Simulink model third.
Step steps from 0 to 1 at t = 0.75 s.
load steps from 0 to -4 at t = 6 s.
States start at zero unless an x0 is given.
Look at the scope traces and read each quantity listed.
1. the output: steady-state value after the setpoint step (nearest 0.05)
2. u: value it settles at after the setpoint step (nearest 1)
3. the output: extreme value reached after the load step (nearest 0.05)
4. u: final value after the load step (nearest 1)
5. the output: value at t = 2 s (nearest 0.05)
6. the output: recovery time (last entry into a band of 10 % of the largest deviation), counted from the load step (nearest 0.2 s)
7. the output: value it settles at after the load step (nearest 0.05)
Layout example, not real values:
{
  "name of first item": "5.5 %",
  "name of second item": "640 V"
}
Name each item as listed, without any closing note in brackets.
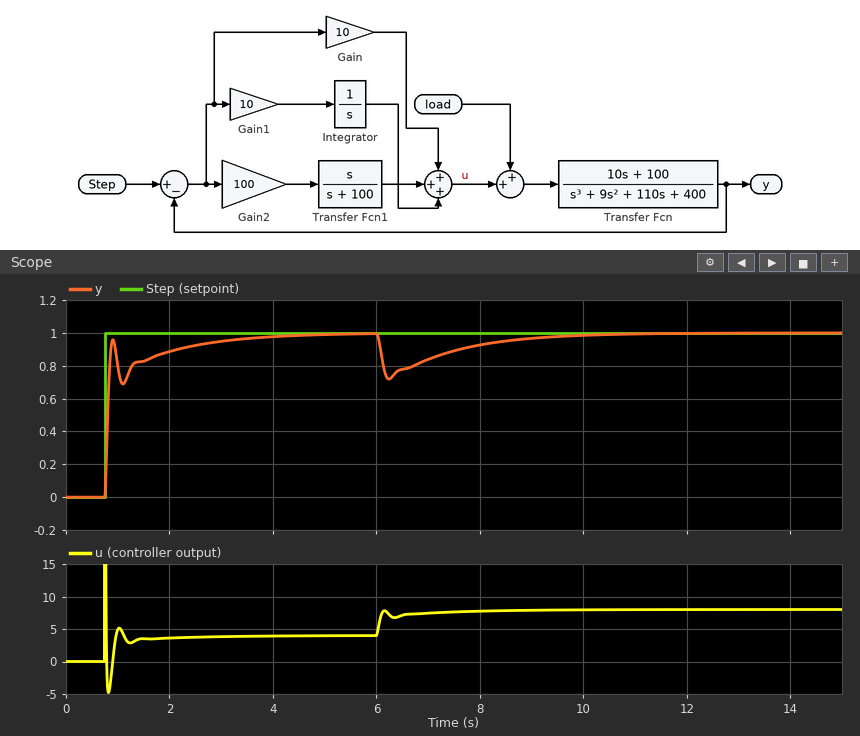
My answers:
{
  "the output: steady-state value after the setpoint step": "1.00",
  "u: value it settles at after the setpoint step": "4",
  "the output: extreme value reached after the load step": "0.70",
  "u: final value after the load step": "8",
  "the output: value at t = 2 s": "0.90",
  "the output: recovery time (last entry into a band of 10 % of the largest deviation), counted from the load step": "3.2 s",
  "the output: value it settles at after the load step": "1.00"
}
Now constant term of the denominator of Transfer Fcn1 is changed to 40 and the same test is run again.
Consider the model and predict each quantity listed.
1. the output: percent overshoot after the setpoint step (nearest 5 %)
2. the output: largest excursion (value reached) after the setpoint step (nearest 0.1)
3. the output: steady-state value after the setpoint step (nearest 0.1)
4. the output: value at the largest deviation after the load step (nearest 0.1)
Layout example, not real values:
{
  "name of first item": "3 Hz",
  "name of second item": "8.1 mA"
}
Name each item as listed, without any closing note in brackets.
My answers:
{
  "the output: percent overshoot after the setpoint step": "10 %",
  "the output: largest excursion (value reached) after the setpoint step": "1.1",
  "the output: steady-state value after the setpoint step": "1.0",
  "the output: value at the largest deviation after the load step": "0.8"
}
